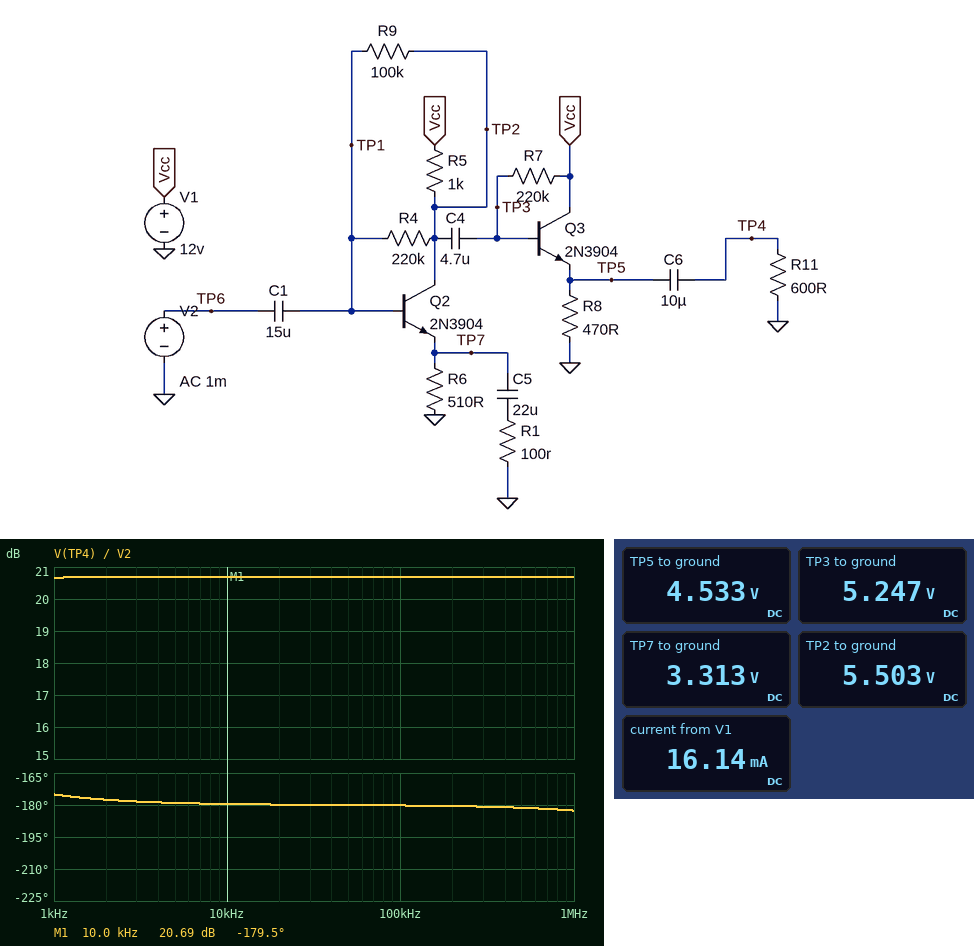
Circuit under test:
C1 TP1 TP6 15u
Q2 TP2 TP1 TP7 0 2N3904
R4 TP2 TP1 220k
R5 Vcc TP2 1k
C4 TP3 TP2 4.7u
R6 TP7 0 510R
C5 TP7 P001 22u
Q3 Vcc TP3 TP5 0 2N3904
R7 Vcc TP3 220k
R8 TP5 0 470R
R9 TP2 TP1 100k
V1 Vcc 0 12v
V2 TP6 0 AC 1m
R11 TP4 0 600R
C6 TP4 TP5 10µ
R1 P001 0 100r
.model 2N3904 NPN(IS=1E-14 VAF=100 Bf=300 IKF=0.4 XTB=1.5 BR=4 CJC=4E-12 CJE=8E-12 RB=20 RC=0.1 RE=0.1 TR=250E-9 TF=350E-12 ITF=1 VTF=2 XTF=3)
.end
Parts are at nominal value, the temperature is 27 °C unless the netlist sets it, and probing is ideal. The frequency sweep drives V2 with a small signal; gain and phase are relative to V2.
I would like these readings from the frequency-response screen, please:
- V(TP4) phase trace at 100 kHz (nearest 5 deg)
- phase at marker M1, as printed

-180 deg
-179.5 deg
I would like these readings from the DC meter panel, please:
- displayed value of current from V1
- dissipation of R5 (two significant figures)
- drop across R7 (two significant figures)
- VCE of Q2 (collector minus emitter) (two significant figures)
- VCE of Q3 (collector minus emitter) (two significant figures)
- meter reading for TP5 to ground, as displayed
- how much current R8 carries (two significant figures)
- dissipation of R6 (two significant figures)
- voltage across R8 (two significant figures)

16.14 mA
42 mW
6.8 V
2.2 V
7.5 V
4.533 V
9.6 mA
22 mW
4.5 V
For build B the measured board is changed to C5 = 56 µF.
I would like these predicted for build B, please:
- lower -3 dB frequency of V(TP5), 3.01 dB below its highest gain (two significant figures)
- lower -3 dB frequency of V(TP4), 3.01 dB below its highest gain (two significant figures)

28 Hz
43 Hz
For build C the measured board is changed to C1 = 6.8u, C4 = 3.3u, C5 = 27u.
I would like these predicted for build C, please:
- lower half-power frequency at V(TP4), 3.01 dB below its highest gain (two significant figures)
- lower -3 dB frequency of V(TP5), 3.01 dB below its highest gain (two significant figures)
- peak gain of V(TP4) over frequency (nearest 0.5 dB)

69 Hz
59 Hz
20.5 dB
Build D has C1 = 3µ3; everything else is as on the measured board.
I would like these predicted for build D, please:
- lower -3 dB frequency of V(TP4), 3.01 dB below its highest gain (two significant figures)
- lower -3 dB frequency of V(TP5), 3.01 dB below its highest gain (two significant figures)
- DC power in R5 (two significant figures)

84 Hz
76 Hz
42 mW
